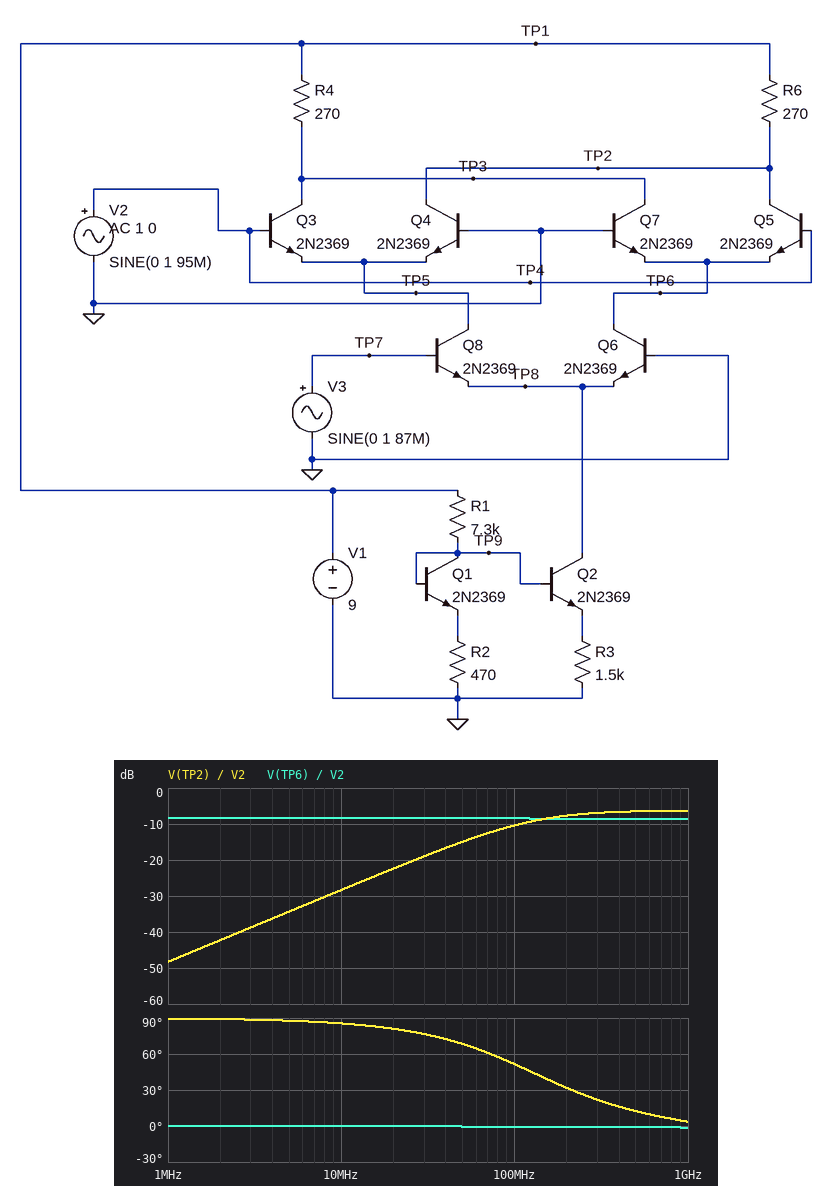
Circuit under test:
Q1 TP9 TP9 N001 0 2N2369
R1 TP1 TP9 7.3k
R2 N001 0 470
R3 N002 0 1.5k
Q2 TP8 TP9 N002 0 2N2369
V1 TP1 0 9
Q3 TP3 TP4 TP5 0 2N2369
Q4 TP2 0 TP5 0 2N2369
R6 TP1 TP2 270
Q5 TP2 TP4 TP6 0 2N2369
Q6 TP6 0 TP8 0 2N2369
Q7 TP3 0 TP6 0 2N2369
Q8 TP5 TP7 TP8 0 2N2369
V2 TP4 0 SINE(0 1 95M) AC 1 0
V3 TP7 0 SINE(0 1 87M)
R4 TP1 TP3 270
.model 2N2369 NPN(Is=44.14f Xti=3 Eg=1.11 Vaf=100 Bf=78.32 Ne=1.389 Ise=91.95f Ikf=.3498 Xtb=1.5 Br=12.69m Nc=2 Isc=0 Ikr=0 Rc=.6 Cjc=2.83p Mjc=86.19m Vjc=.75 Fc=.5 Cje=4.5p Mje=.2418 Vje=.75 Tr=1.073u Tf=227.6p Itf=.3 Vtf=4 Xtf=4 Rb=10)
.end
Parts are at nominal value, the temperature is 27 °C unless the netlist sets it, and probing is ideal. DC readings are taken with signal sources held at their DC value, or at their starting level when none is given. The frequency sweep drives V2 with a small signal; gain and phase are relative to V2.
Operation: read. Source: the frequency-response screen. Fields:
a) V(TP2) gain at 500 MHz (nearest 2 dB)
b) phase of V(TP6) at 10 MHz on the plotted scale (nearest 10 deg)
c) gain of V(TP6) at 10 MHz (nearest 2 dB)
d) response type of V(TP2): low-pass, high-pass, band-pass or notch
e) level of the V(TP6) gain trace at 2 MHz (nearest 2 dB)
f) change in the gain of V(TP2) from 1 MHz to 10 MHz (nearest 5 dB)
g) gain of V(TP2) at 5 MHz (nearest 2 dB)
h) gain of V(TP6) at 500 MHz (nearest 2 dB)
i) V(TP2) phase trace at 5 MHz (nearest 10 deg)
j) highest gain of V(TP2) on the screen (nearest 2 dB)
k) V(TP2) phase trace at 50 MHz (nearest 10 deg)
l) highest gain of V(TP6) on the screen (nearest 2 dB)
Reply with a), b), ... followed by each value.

a) -6 dB
b) 0 deg
c) -8 dB
d) high-pass
e) -8 dB
f) 20 dB
g) -34 dB
h) -8 dB
i) 90 deg
j) -6 dB
k) 70 deg
l) -8 dB
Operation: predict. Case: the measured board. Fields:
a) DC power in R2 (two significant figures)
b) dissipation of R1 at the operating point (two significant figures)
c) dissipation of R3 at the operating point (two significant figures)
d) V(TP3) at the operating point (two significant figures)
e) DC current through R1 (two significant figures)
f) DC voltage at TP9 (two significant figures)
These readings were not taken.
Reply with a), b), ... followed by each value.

a) 320 µW
b) 8.8 mW
c) 110 µW
d) 9.0 V
e) 1.1 mA
f) 1.0 V
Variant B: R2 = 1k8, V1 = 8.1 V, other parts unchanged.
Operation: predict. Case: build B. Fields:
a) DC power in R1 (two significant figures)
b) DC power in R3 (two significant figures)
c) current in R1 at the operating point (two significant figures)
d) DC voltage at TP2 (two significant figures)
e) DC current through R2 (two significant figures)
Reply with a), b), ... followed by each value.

a) 6.2 mW
b) 380 µW
c) 920 µA
d) 8.1 V
e) 420 µA
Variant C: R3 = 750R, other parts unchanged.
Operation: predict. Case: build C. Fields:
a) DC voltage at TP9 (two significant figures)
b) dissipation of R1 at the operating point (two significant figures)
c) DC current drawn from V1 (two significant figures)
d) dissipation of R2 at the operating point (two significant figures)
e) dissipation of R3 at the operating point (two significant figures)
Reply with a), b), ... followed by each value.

a) 920 mV
b) 8.9 mW
c) 1.1 mA
d) 210 µW
e) 140 µW
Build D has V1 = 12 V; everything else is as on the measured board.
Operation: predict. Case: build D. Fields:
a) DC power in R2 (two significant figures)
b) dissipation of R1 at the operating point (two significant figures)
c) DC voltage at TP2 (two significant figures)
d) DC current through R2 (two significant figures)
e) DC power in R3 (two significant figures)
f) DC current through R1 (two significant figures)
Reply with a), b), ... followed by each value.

a) 590 µW
b) 16 mW
c) 12 V
d) 1.1 mA
e) 200 µW
f) 1.5 mA
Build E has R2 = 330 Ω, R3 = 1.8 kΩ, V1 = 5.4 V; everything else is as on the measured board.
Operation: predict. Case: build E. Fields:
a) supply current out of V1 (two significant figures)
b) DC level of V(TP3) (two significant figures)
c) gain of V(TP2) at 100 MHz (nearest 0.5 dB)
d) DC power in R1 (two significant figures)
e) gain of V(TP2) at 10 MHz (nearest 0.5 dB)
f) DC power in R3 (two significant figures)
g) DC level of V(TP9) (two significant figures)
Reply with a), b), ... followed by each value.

a) 630 µA
b) 5.4 V
c) -10.0 dB
d) 2.9 mW
e) -28.0 dB
f) 24 µW
g) 770 mV
